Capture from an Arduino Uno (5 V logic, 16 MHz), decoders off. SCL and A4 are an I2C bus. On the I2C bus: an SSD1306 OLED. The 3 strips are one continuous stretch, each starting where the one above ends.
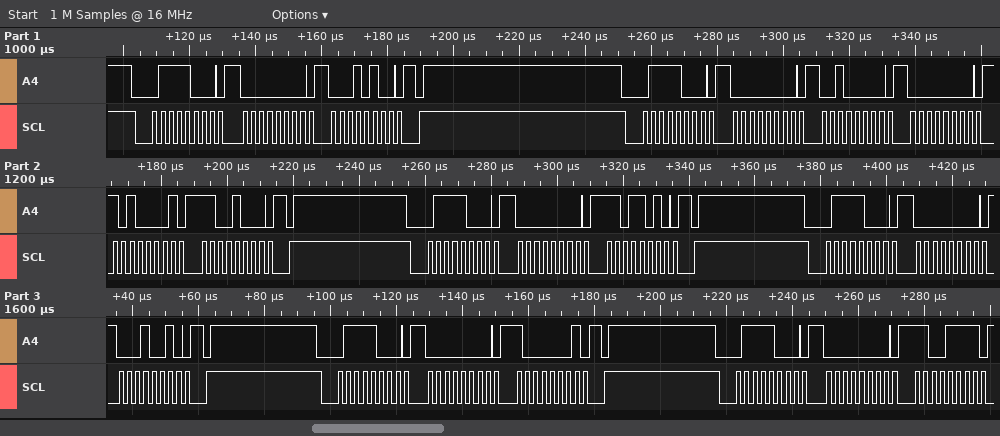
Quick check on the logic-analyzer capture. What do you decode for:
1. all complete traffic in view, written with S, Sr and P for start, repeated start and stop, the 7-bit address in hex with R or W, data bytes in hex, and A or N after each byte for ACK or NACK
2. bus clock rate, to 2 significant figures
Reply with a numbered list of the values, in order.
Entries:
1. S 3CW A 00 A 14 A P S 3CW A 00 A 20 A 00 A A1 A C8 A P S 3CW A 00 A DA A P S 3CW A 00 A 12 A P S 3CW A 00 A 81 A P S 3CW A 00 A CF A
2. 400 kHz
